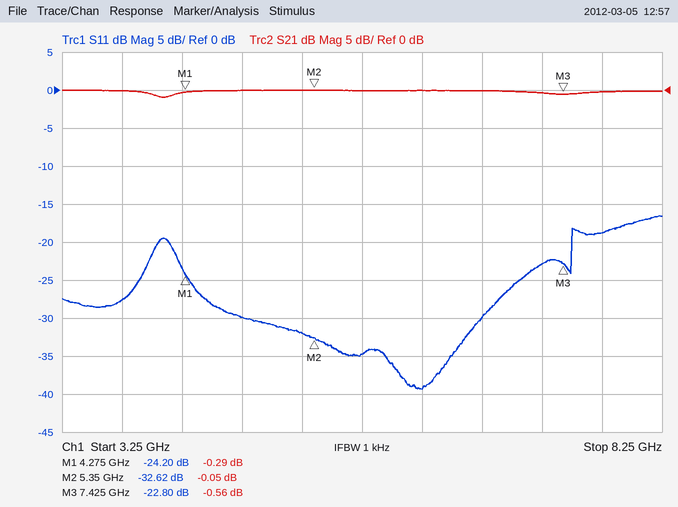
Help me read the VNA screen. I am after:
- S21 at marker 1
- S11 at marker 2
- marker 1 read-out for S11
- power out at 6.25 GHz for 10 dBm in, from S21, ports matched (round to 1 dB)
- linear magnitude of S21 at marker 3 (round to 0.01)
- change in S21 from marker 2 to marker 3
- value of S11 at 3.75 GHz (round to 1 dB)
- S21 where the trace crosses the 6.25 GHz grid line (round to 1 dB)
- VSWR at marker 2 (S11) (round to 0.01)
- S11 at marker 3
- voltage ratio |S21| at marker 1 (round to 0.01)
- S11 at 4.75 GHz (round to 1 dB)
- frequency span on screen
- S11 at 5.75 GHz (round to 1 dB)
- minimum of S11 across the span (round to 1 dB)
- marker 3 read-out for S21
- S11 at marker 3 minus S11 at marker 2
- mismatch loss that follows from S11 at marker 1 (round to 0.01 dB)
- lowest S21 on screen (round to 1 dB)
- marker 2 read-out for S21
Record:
-0.29 dB
-32.62 dB
-24.20 dB
10 dBm
0.94
-0.51 dB
-28 dB
0 dB
1.05
-22.80 dB
0.97
-30 dB
5 GHz
-35 dB
-39 dB
-0.56 dB
9.82 dB
0.02 dB
-1 dB
-0.05 dB
